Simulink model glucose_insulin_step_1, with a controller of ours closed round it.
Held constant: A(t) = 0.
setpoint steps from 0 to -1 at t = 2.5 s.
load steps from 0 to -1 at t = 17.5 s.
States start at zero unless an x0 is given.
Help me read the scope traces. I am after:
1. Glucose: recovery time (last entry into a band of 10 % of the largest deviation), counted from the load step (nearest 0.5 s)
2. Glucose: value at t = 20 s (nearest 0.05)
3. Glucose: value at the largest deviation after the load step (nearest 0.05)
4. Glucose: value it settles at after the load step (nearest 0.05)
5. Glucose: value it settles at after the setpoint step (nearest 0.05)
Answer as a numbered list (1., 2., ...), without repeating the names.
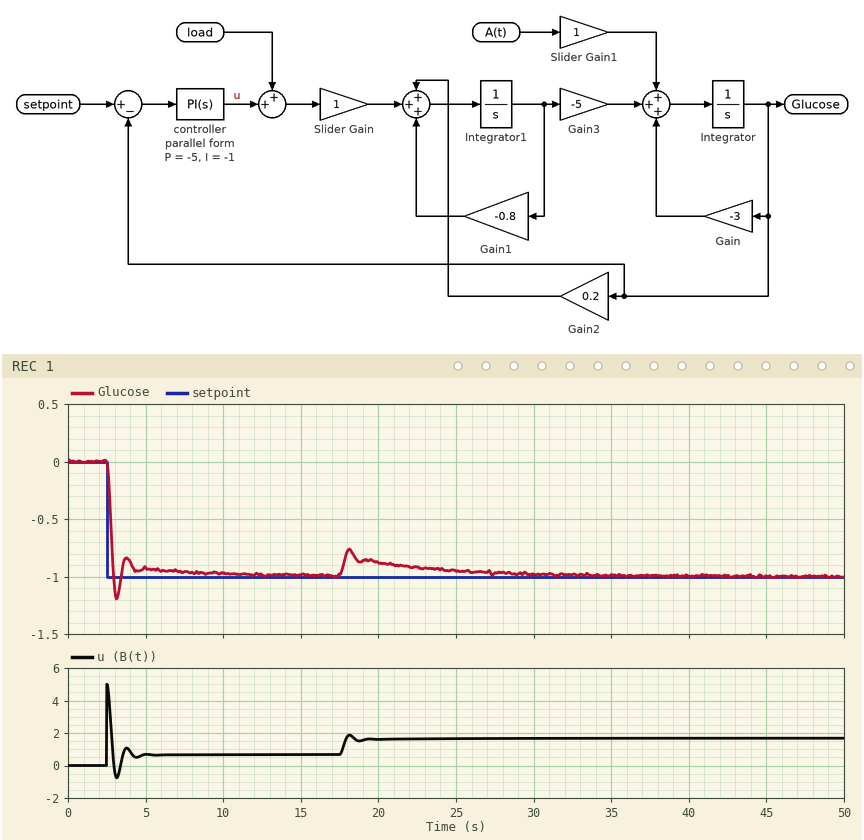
1. 12.0 s
2. -0.90
3. -0.75
4. -1.00
5. -1.00
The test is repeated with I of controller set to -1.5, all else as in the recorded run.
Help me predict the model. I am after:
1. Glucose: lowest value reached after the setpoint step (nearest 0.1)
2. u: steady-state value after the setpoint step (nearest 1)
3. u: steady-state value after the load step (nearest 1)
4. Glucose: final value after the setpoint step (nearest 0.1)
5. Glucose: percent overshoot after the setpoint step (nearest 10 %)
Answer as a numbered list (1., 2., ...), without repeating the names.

1. -1.2
2. 1
3. 2
4. -1.0
5. 20 %
